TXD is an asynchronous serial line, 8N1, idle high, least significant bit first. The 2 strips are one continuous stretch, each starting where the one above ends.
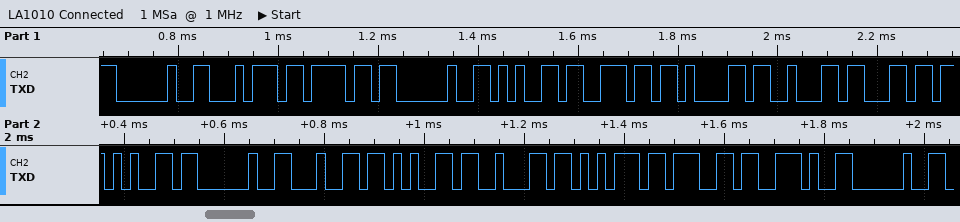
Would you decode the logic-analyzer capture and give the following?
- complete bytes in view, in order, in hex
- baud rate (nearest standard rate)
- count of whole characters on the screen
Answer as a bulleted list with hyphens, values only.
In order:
- 20 74 6F 20 65 6E 61 62 6C 65 20 64 65 62 75 67 2E 20
- 57600 baud
- 18
